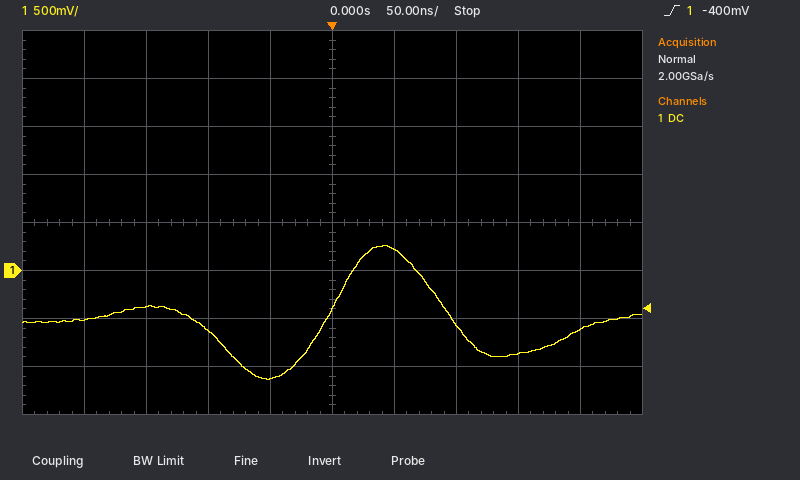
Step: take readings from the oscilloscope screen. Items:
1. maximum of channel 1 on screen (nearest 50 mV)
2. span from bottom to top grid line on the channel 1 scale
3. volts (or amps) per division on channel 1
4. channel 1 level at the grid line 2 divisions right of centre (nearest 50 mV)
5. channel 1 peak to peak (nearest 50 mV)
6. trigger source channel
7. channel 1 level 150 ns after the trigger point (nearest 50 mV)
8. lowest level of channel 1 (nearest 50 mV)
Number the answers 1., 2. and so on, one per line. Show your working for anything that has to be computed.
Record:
1. 250 mV
2. 4 V
3. 500 mV
4. -550 mV
5. 250 mV − (-1.15 V) = 1.40 V
6. channel 1
7. -850 mV
8. -1.15 V
